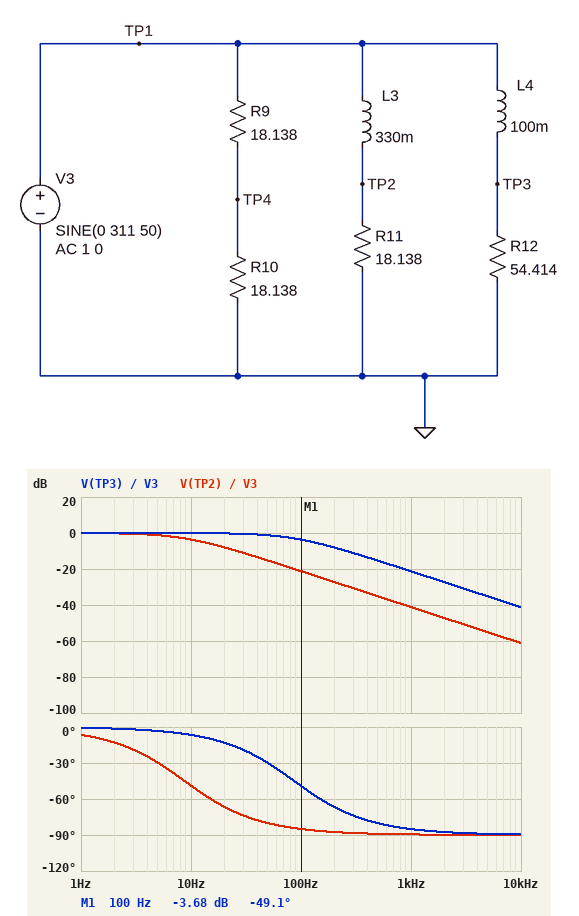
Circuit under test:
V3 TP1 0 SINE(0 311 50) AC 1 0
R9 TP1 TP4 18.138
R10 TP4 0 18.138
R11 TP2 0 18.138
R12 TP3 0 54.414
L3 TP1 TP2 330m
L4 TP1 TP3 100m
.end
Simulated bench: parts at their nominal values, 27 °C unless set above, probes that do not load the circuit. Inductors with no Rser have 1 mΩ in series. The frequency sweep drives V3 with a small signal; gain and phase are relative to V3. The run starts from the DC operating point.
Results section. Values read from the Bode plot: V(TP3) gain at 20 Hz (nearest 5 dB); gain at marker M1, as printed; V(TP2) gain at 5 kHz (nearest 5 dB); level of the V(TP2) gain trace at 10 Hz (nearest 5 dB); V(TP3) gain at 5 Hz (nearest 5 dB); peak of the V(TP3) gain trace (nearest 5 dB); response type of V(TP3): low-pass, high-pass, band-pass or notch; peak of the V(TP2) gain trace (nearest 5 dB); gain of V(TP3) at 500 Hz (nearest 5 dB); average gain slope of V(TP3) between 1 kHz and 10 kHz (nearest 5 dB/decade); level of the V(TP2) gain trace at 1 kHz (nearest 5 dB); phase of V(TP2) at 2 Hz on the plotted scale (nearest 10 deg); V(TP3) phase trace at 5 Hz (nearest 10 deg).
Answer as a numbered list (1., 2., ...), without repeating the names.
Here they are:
1. 0 dB
2. -3.68 dB
3. -55 dB
4. -5 dB
5. 0 dB
6. 0 dB
7. low-pass
8. 0 dB
9. -15 dB
10. -20 dB/decade
11. -40 dB
12. -10 deg
13. 0 deg
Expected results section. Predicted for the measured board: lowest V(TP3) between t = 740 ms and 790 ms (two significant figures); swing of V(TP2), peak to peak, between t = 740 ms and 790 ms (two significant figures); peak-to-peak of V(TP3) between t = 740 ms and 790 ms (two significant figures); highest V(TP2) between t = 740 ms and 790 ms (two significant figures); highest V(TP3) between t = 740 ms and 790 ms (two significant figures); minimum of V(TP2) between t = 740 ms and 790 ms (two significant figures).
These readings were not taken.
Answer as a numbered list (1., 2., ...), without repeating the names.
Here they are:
1. -270 V
2. 110 V
3. 540 V
4. 54 V
5. 270 V
6. -54 V
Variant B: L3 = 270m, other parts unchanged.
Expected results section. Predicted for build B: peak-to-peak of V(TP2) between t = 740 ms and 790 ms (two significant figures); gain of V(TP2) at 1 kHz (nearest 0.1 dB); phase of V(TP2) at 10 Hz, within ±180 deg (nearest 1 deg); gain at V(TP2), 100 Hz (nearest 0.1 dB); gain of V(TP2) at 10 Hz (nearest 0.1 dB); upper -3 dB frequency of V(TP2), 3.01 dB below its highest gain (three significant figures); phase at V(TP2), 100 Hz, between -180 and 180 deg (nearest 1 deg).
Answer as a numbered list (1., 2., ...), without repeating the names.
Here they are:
1. 130 V
2. -39.4 dB
3. -43 deg
4. -19.5 dB
5. -2.7 dB
6. 10.7 Hz
7. -84 deg
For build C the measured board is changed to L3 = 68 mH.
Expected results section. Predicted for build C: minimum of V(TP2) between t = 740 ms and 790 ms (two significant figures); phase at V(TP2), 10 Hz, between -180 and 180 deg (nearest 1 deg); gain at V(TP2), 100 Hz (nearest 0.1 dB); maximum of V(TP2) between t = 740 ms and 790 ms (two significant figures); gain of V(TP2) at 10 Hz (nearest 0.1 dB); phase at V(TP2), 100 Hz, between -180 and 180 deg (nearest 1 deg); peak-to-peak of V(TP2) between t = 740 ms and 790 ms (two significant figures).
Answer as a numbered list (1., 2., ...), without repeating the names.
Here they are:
1. -200 V
2. -13 deg
3. -8.2 dB
4. 200 V
5. -0.2 dB
6. -67 deg
7. 400 V
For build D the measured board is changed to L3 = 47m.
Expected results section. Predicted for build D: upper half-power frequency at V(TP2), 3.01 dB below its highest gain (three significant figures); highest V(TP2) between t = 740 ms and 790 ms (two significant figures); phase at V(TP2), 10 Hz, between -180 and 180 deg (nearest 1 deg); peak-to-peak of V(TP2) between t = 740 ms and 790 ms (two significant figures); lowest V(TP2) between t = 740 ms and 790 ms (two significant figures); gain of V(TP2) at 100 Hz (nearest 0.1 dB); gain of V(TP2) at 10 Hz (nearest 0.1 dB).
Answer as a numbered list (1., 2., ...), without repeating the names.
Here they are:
1. 61.4 Hz
2. 240 V
3. -9 deg
4. 480 V
5. -240 V
6. -5.6 dB
7. -0.1 dB
